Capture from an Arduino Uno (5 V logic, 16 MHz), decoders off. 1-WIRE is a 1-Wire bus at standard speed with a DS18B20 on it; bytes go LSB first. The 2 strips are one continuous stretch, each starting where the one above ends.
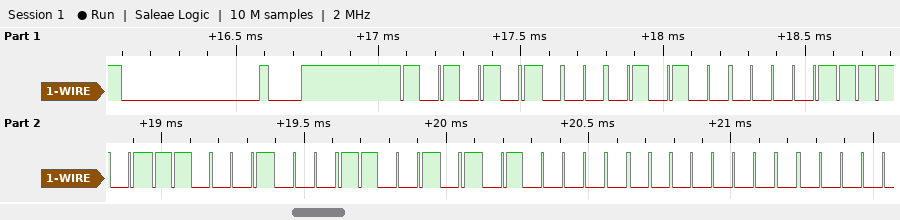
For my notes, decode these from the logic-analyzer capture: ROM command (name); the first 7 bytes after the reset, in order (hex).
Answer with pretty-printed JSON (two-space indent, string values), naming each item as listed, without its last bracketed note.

{
  "ROM command": "Match ROM",
  "the first 7 bytes after the reset, in order": "55 28 F0 8E 98 0A 00"
}
